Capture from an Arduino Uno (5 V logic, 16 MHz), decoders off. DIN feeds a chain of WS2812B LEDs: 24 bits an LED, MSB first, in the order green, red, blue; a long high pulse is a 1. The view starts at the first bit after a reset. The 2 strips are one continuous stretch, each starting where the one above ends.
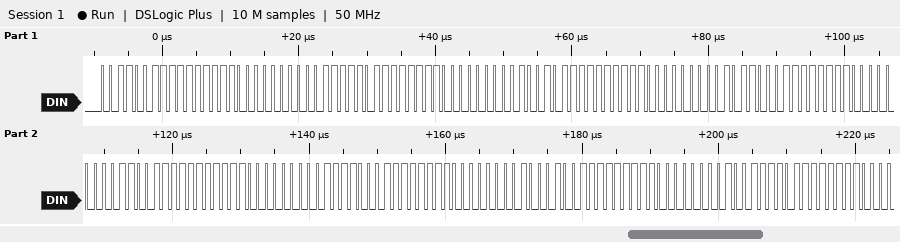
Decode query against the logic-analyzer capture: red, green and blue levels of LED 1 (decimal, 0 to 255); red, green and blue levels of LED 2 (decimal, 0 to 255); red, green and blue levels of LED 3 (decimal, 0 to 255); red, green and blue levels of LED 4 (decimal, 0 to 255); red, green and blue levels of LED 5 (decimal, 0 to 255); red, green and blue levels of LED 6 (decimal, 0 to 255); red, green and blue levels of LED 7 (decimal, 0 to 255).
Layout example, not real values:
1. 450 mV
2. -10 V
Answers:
1. 255, 51, 0
2. 255, 62, 0
3. 255, 75, 0
4. 255, 88, 0
5. 255, 103, 0
6. 255, 120, 0
7. 255, 137, 0
